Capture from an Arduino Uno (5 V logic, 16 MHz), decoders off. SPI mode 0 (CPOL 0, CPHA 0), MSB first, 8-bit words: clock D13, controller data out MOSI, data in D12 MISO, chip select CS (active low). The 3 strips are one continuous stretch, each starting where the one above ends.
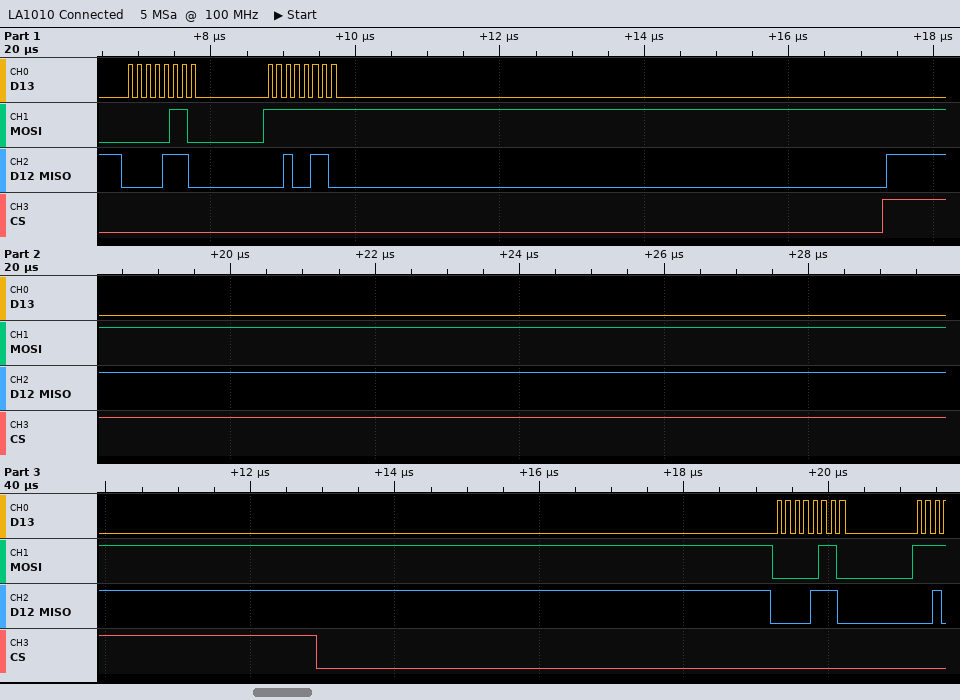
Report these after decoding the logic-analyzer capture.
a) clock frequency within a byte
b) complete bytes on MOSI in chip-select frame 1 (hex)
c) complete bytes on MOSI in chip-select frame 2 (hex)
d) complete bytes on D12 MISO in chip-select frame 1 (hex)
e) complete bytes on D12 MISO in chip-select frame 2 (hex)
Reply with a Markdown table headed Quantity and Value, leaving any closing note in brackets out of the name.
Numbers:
| Quantity | Value |
|---|---|
| clock frequency within a byte | 8 MHz |
| complete bytes on MOSI in chip-select frame 1 | 0x06 0xFF |
| complete bytes on MOSI in chip-select frame 2 | 0x06 |
| complete bytes on D12 MISO in chip-select frame 1 | 0x0E 0x26 |
| complete bytes on D12 MISO in chip-select frame 2 | 0x0E |
